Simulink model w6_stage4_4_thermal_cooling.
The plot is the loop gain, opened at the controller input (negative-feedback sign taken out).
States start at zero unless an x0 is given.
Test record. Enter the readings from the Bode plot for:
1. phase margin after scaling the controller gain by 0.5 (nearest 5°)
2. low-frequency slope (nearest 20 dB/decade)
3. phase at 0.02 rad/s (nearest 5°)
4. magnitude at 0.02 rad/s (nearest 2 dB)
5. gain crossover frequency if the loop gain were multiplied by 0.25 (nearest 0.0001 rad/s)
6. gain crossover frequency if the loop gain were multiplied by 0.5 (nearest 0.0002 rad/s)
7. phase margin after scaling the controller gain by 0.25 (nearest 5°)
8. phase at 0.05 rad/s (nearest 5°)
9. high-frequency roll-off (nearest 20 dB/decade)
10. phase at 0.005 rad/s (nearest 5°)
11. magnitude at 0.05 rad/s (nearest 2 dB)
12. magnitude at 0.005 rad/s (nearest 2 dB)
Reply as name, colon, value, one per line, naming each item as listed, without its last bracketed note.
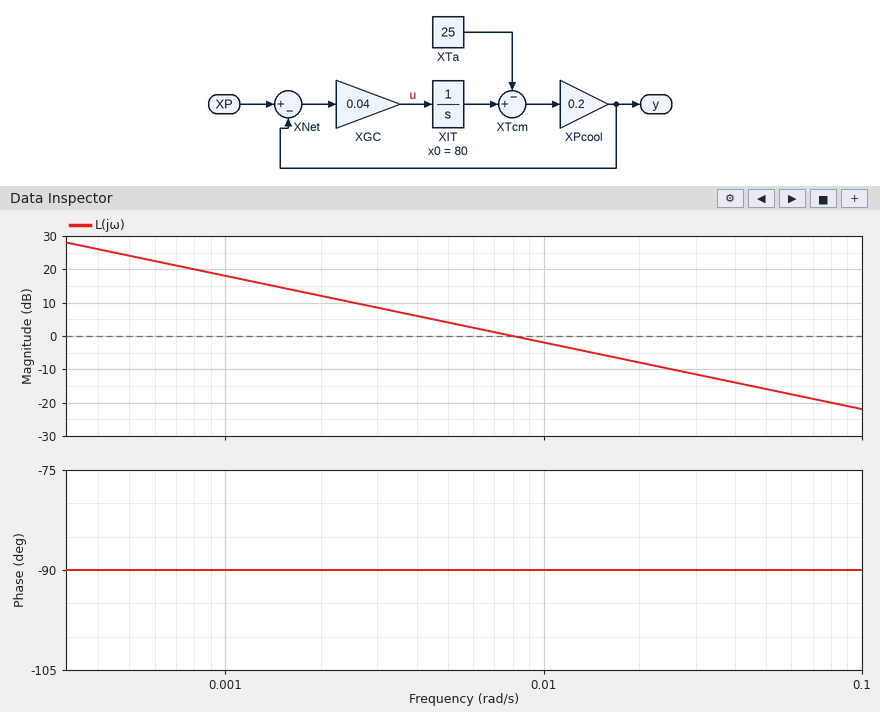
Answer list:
phase margin after scaling the controller gain by 0.5: 90°
low-frequency slope: -20 dB/decade
phase at 0.02 rad/s: -90°
magnitude at 0.02 rad/s: -8 dB
gain crossover frequency if the loop gain were multiplied by 0.25: 0.0020 rad/s
gain crossover frequency if the loop gain were multiplied by 0.5: 0.0040 rad/s
phase margin after scaling the controller gain by 0.25: 90°
phase at 0.05 rad/s: -90°
high-frequency roll-off: -20 dB/decade
phase at 0.005 rad/s: -90°
magnitude at 0.05 rad/s: -16 dB
magnitude at 0.005 rad/s: 4 dB
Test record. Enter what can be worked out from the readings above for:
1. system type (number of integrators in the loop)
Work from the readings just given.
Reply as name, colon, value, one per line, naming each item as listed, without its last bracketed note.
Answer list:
system type: 1
